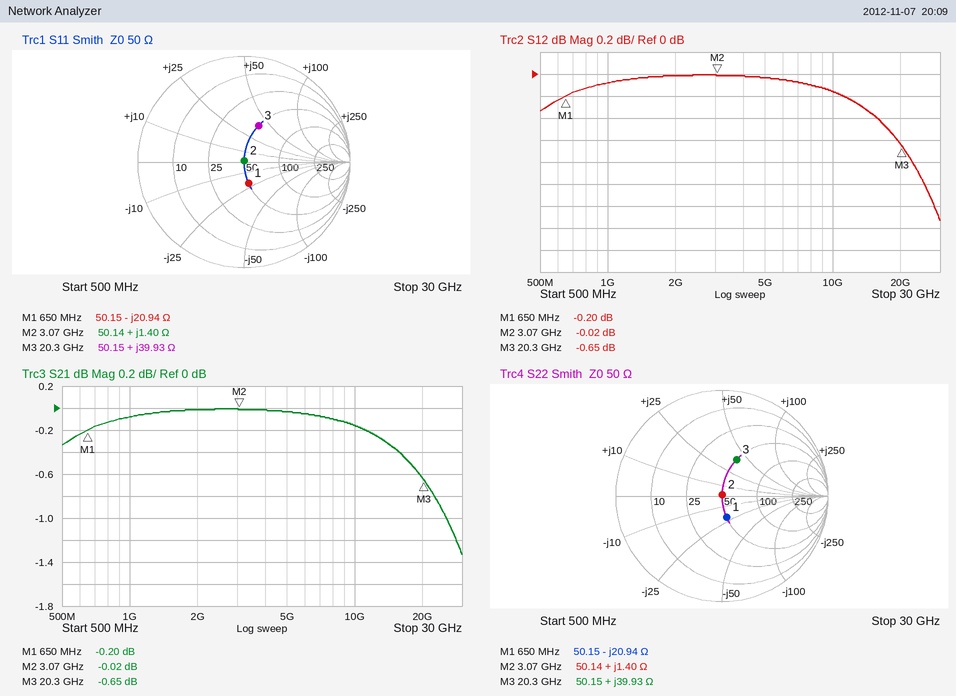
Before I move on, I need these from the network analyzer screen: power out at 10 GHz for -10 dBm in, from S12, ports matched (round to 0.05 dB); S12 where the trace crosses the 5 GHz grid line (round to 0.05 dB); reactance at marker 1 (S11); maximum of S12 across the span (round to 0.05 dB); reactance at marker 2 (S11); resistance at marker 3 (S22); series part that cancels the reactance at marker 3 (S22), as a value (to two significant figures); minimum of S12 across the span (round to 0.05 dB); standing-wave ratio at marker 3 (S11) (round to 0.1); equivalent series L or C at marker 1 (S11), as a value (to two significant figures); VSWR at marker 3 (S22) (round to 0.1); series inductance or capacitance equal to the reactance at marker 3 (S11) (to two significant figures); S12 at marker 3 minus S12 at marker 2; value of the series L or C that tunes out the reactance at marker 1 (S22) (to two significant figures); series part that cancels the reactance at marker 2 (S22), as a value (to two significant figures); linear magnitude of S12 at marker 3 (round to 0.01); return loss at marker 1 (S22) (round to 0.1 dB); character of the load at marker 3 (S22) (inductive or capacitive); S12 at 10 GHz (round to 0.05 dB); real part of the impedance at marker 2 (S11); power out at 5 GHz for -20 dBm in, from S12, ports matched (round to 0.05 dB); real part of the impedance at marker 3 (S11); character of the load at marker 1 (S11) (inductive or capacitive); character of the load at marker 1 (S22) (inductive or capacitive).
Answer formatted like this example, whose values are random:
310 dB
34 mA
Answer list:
-10.15 dBm
-0.05 dB
-20.94 Ω
0.00 dB
+1.40 Ω
50.15 Ω
200 fF
-1.35 dB
2.2
12 pF
2.2
310 pH
-0.63 dB
5.1 nH
37 pF
0.93
13.8 dB
inductive
-0.15 dB
50.14 Ω
-20.05 dBm
50.15 Ω
capacitive
capacitive
